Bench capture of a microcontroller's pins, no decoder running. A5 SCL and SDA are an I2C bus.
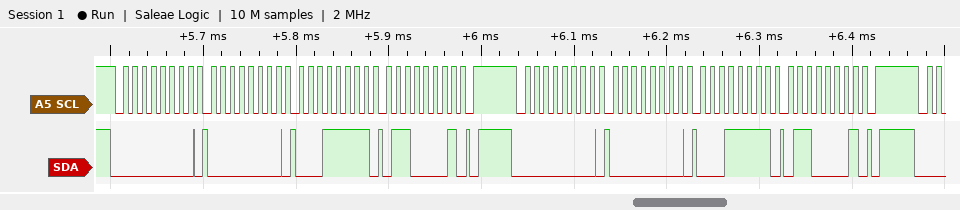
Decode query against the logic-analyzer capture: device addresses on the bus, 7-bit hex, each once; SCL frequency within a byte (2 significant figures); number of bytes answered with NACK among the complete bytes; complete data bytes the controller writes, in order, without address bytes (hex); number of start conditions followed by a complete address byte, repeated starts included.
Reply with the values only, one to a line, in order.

0x00
100 kHz
0
00 1F 61 00 1F 61
2
